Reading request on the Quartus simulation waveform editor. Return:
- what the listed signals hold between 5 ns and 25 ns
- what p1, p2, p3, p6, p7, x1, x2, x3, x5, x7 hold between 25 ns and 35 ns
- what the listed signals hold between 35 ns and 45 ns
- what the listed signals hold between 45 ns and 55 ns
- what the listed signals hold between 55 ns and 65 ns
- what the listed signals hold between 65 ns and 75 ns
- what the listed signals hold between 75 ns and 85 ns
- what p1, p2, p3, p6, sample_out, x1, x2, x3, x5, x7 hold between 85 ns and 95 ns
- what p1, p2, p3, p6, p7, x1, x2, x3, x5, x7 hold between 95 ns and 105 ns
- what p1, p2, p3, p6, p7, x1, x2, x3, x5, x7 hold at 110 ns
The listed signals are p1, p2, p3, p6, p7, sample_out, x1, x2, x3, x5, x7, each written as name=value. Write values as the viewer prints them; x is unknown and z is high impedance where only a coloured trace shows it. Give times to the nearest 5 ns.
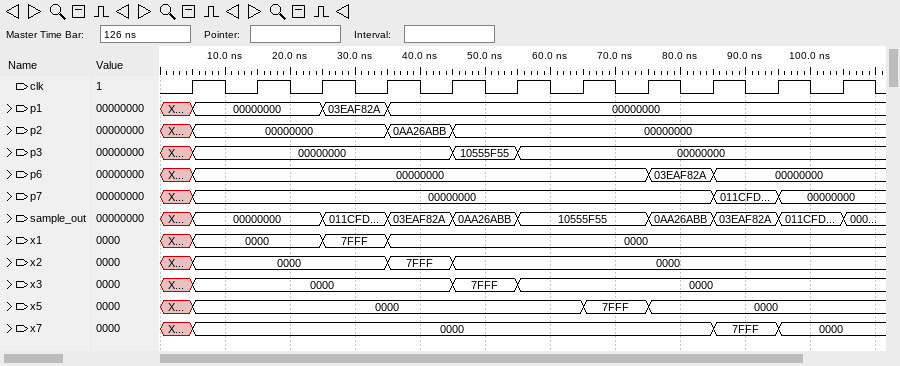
p1=00000000, p2=00000000, p3=00000000, p6=00000000, p7=00000000, sample_out=00000000, x1=0000, x2=0000, x3=0000, x5=0000, x7=0000
p1=03EAF82A, p2=00000000, p3=00000000, p6=00000000, p7=00000000, x1=7FFF, x2=0000, x3=0000, x5=0000, x7=0000
p1=00000000, p2=0AA26ABB, p3=00000000, p6=00000000, p7=00000000, sample_out=03EAF82A, x1=0000, x2=7FFF, x3=0000, x5=0000, x7=0000
p1=00000000, p2=00000000, p3=10555F55, p6=00000000, p7=00000000, sample_out=0AA26ABB, x1=0000, x2=0000, x3=7FFF, x5=0000, x7=0000
p1=00000000, p2=00000000, p3=00000000, p6=00000000, p7=00000000, sample_out=10555F55, x1=0000, x2=0000, x3=0000, x5=0000, x7=0000
p1=00000000, p2=00000000, p3=00000000, p6=00000000, p7=00000000, sample_out=10555F55, x1=0000, x2=0000, x3=0000, x5=7FFF, x7=0000
p1=00000000, p2=00000000, p3=00000000, p6=03EAF82A, p7=00000000, sample_out=0AA26ABB, x1=0000, x2=0000, x3=0000, x5=0000, x7=0000
p1=00000000, p2=00000000, p3=00000000, p6=00000000, sample_out=03EAF82A, x1=0000, x2=0000, x3=0000, x5=0000, x7=7FFF
p1=00000000, p2=00000000, p3=00000000, p6=00000000, p7=00000000, x1=0000, x2=0000, x3=0000, x5=0000, x7=0000
p1=00000000, p2=00000000, p3=00000000, p6=00000000, p7=00000000, x1=0000, x2=0000, x3=0000, x5=0000, x7=0000
